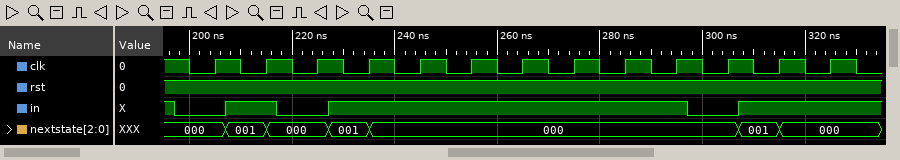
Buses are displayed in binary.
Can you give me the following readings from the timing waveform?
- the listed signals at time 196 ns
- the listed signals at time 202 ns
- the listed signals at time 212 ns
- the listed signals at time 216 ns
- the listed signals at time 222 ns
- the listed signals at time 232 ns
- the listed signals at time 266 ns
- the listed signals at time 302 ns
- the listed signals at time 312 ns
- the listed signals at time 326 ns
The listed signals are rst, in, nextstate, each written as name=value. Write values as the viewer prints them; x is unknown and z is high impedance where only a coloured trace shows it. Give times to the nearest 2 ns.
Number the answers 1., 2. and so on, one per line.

1. rst=1, in=1, nextstate=000
2. rst=1, in=0, nextstate=000
3. rst=1, in=1, nextstate=001
4. rst=1, in=1, nextstate=000
5. rst=1, in=0, nextstate=000
6. rst=1, in=1, nextstate=001
7. rst=1, in=1, nextstate=000
8. rst=1, in=0, nextstate=000
9. rst=1, in=1, nextstate=001
10. rst=1, in=1, nextstate=000
